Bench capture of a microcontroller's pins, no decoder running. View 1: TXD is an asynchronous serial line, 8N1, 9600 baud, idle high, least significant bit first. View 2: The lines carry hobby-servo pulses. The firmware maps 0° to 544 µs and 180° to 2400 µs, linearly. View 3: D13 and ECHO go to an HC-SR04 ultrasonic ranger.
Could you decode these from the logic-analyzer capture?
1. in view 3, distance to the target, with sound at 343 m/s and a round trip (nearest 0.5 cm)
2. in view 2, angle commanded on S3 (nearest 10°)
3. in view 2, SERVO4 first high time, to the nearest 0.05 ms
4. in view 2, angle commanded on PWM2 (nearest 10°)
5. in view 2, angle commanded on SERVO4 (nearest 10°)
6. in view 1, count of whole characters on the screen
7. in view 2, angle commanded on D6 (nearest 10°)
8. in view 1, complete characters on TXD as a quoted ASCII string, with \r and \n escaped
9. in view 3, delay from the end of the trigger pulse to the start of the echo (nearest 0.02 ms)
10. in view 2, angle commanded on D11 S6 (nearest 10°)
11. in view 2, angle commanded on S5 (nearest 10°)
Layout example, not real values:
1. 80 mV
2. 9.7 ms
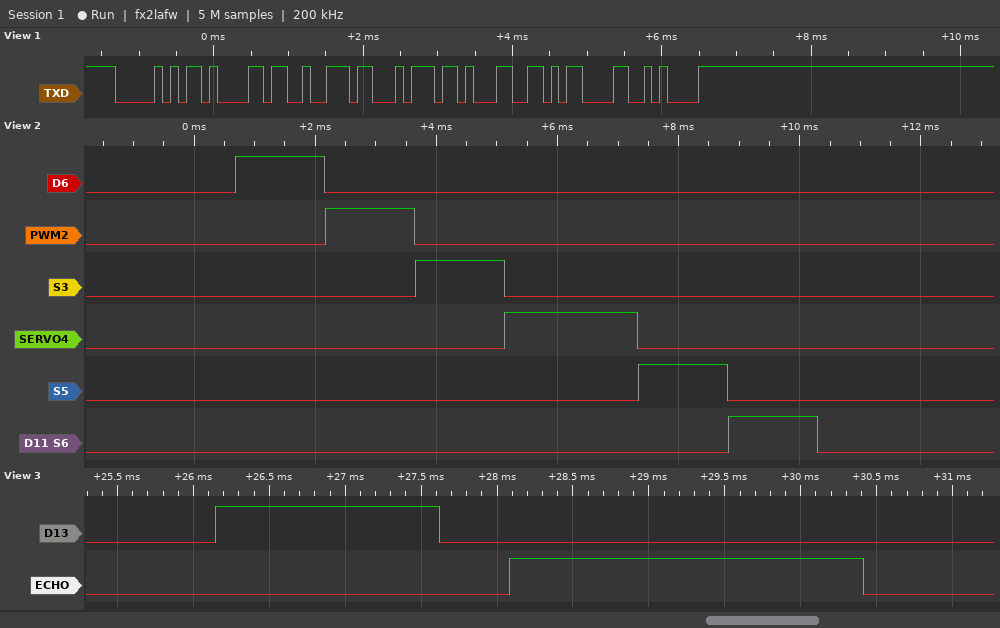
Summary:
1. 40 cm
2. 90°
3. 2.20 ms
4. 90°
5. 160°
6. 7
7. 90°
8. "Part1\r\n"
9. 0.46 ms
10. 90°
11. 90°
